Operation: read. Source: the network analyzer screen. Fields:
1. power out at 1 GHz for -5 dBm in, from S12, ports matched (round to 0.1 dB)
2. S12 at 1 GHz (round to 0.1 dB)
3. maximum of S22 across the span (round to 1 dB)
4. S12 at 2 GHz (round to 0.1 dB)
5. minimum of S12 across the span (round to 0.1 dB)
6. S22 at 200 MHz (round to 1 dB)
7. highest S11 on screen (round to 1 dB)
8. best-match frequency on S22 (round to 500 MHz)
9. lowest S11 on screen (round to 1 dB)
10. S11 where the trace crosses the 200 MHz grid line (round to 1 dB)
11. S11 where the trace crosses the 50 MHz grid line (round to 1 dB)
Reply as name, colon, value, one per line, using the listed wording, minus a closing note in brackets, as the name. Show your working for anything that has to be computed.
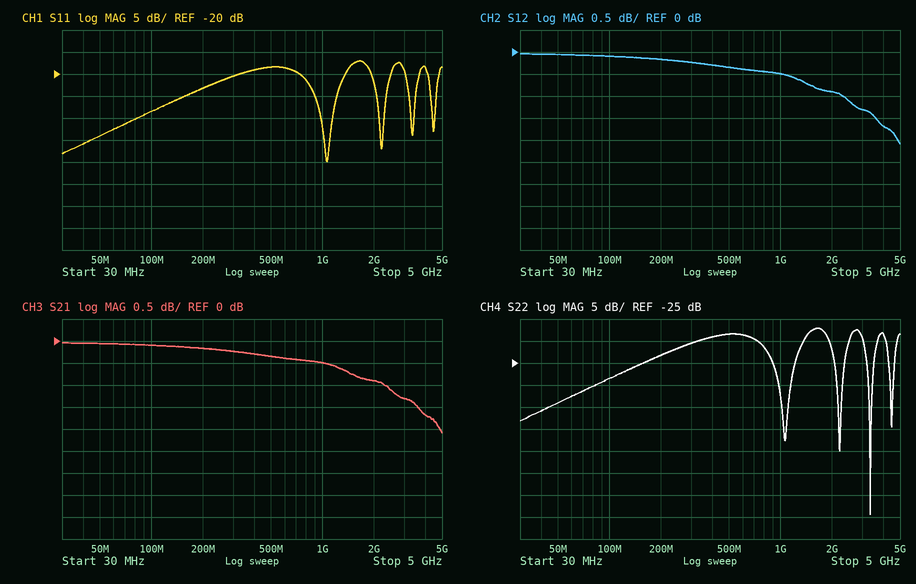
power out at 1 GHz for -5 dBm in, from S12, ports matched: -5 dBm + (-0.5 dB) = -5.5 dBm
S12 at 1 GHz: -0.5 dB
maximum of S22 across the span: -17 dB
S12 at 2 GHz: -0.9 dB
minimum of S12 across the span: -2.1 dB
S22 at 200 MHz: -23 dB
highest S11 on screen: -17 dB
best-match frequency on S22: 3.5 GHz
lowest S11 on screen: -40 dB
S11 where the trace crosses the 200 MHz grid line: -23 dB
S11 where the trace crosses the 50 MHz grid line: -34 dB
